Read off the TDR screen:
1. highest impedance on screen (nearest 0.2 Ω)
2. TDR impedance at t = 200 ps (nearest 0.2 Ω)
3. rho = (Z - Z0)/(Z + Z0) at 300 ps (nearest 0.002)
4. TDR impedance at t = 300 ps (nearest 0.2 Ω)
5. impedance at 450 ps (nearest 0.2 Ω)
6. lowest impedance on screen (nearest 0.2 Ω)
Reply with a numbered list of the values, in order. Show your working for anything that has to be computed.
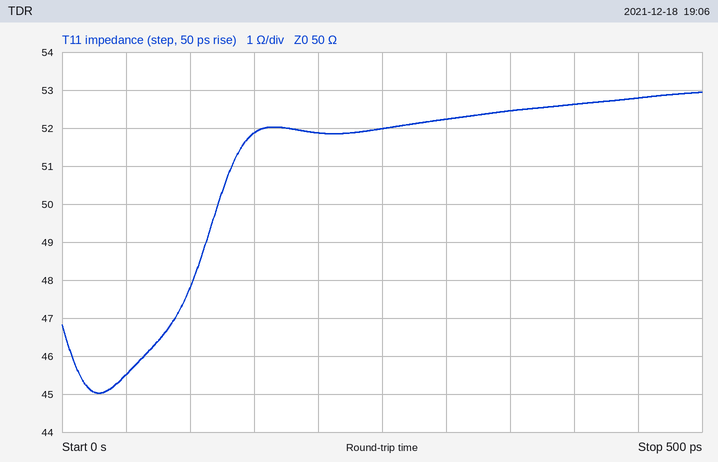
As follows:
1. 53.0 Ω
2. 51.8 Ω
3. (52.2 − 50)/(52.2 + 50) ≈ +0.022
4. 52.2 Ω
5. 52.8 Ω
6. 45.0 Ω
